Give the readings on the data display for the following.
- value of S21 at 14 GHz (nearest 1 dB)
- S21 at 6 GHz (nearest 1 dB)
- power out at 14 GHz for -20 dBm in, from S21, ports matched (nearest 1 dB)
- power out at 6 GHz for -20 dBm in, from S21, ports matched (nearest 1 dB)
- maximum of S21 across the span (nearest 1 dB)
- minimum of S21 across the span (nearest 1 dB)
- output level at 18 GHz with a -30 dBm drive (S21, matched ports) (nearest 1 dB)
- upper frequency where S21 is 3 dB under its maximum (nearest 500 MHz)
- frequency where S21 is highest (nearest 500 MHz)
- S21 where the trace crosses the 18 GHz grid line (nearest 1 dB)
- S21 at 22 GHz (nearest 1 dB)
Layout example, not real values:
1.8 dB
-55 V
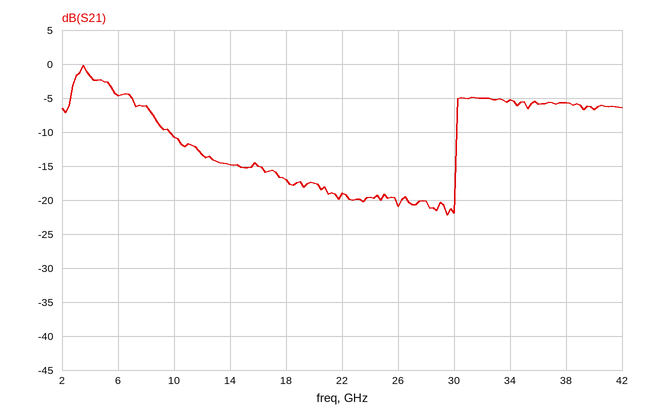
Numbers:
-15 dB
-5 dB
-35 dBm
-25 dBm
0 dB
-22 dB
-47 dBm
5.5 GHz
3.5 GHz
-17 dB
-19 dB
